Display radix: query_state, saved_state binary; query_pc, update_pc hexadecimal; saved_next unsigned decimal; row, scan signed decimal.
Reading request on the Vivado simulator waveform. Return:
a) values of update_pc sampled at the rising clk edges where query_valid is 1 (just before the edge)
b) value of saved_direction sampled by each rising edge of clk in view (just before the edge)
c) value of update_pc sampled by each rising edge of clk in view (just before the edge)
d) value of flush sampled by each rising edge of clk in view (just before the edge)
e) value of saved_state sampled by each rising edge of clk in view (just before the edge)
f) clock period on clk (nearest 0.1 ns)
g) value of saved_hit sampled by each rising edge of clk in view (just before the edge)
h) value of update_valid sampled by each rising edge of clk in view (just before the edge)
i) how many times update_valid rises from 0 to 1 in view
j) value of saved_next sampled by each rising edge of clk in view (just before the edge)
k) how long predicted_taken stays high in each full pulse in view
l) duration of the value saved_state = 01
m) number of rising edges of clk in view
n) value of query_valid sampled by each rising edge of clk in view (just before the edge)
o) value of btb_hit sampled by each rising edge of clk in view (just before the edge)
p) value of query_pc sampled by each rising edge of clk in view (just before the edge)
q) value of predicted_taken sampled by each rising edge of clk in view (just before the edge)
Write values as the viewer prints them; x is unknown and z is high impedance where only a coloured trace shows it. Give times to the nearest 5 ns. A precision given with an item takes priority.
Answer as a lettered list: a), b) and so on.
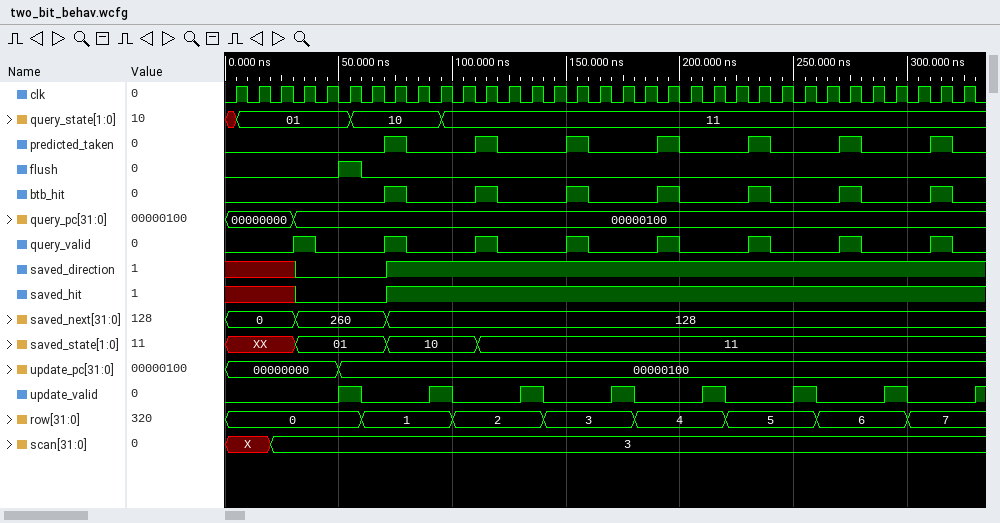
a) 00000000, 00000100, 00000100, 00000100, 00000100, 00000100, 00000100, 00000100
b) x x x 0 0 0 0 1 1 1 1 1 1 1 1 1 1 1 1 1 1 1 1 1 1 1 1 1 1 1 1 1 1
c) 00000000, 00000000, 00000000, 00000000, 00000000, 00000100, 00000100, 00000100, 00000100, 00000100, 00000100, 00000100, 00000100, 00000100, 00000100, 00000100, 00000100, 00000100, 00000100, 00000100, 00000100, 00000100, 00000100, 00000100, 00000100, 00000100, 00000100, 00000100, 00000100, 00000100, 00000100, 00000100, 00000100
d) 0 0 0 0 0 1 0 0 0 0 0 0 0 0 0 0 0 0 0 0 0 0 0 0 0 0 0 0 0 0 0 0 0
e) XX, XX, XX, 01, 01, 01, 01, 10, 10, 10, 10, 11, 11, 11, 11, 11, 11, 11, 11, 11, 11, 11, 11, 11, 11, 11, 11, 11, 11, 11, 11, 11, 11
f) 10 ns
g) x x x 0 0 0 0 1 1 1 1 1 1 1 1 1 1 1 1 1 1 1 1 1 1 1 1 1 1 1 1 1 1
h) 0 0 0 0 0 1 0 0 0 1 0 0 0 1 0 0 0 1 0 0 0 1 0 0 0 1 0 0 0 1 0 0 0
i) 8
j) 0, 0, 0, 260, 260, 260, 260, 128, 128, 128, 128, 128, 128, 128, 128, 128, 128, 128, 128, 128, 128, 128, 128, 128, 128, 128, 128, 128, 128, 128, 128, 128, 128
k) 10 ns, 10 ns, 10 ns, 10 ns, 10 ns, 10 ns, 10 ns
l) 40 ns
m) 33
n) 0 0 0 1 0 0 0 1 0 0 0 1 0 0 0 1 0 0 0 1 0 0 0 1 0 0 0 1 0 0 0 1 0
o) 0 0 0 0 0 0 0 1 0 0 0 1 0 0 0 1 0 0 0 1 0 0 0 1 0 0 0 1 0 0 0 1 0
p) 00000000, 00000000, 00000000, 00000100, 00000100, 00000100, 00000100, 00000100, 00000100, 00000100, 00000100, 00000100, 00000100, 00000100, 00000100, 00000100, 00000100, 00000100, 00000100, 00000100, 00000100, 00000100, 00000100, 00000100, 00000100, 00000100, 00000100, 00000100, 00000100, 00000100, 00000100, 00000100, 00000100
q) 0 0 0 0 0 0 0 1 0 0 0 1 0 0 0 1 0 0 0 1 0 0 0 1 0 0 0 1 0 0 0 1 0
